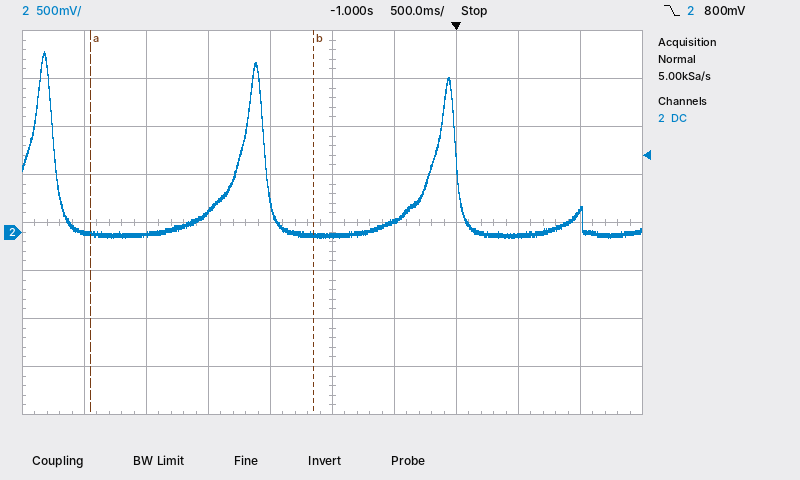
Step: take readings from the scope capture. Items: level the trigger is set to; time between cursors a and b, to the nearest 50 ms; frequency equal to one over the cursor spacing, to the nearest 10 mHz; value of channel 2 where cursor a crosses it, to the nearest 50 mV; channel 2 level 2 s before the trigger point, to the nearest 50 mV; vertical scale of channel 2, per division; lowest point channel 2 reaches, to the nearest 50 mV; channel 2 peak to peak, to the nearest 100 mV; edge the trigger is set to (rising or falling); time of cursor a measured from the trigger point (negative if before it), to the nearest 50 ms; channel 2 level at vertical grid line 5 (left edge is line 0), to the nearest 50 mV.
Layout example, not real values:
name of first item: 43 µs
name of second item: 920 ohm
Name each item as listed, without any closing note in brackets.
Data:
level the trigger is set to: 800 mV
time between cursors a and b, to the nearest 50 ms: 1.80 s
frequency equal to one over the cursor spacing, to the nearest 10 mHz: 560 mHz
value of channel 2 where cursor a crosses it, to the nearest 50 mV: 0 mV
channel 2 level 2 s before the trigger point, to the nearest 50 mV: 200 mV
vertical scale of channel 2, per division: 500 mV
lowest point channel 2 reaches, to the nearest 50 mV: -50 mV
channel 2 peak to peak, to the nearest 100 mV: 1.90 V
edge the trigger is set to: falling
time of cursor a measured from the trigger point (negative if before it), to the nearest 50 ms: -2.95 s
channel 2 level at vertical grid line 5 (left edge is line 0), to the nearest 50 mV: -50 mV
